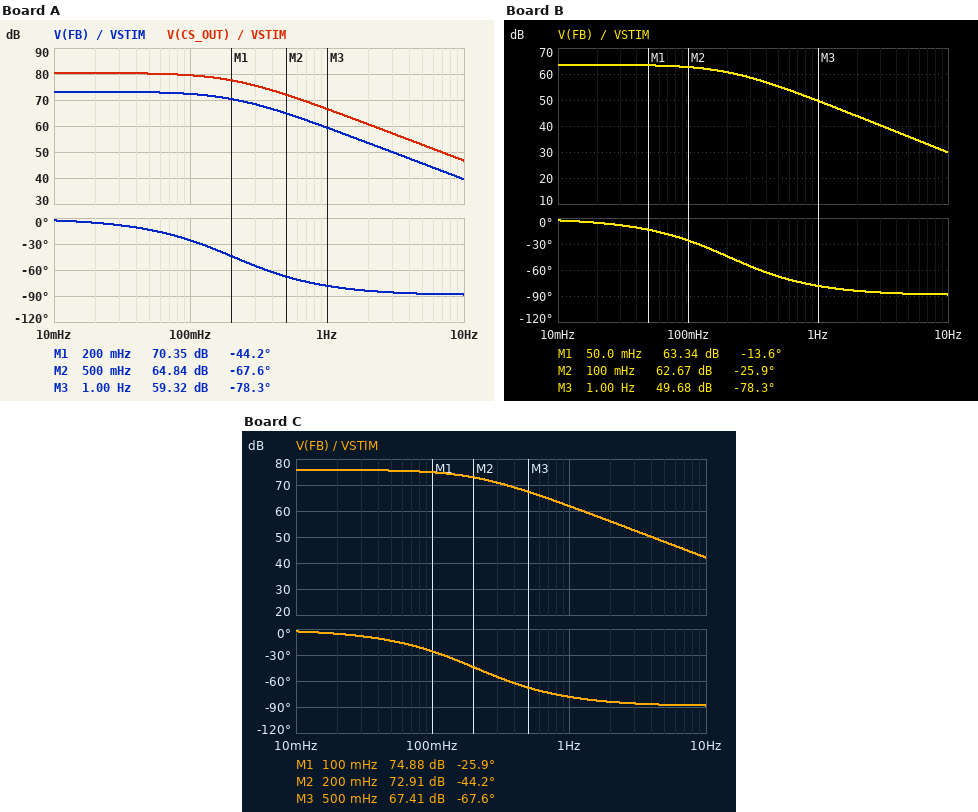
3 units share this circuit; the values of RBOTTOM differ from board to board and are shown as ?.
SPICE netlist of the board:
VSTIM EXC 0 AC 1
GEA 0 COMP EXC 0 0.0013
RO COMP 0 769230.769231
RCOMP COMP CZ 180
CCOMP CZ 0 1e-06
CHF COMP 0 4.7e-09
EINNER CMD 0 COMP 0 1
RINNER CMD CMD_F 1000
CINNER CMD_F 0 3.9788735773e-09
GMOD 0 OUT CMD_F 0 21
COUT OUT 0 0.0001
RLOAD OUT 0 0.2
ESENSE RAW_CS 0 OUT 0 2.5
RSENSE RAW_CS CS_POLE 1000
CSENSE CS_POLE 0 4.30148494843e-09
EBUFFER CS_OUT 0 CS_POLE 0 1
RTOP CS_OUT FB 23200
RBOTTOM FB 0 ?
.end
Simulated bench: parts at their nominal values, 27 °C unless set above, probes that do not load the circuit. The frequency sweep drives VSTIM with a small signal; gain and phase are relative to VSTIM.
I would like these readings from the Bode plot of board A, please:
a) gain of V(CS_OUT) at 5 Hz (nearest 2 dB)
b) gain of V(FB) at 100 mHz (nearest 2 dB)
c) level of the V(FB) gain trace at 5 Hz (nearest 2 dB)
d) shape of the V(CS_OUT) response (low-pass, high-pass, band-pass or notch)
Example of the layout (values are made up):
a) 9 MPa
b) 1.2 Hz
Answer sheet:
a) 52 dB
b) 72 dB
c) 46 dB
d) low-pass
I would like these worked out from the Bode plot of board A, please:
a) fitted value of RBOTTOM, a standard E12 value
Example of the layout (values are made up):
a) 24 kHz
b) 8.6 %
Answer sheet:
a) 18 kΩ
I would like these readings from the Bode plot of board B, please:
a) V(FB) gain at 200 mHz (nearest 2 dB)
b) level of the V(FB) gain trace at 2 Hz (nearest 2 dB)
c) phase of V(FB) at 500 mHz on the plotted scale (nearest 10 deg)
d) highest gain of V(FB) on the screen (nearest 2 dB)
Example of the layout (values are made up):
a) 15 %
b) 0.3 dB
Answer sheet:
a) 60 dB
b) 44 dB
c) -70 deg
d) 64 dB
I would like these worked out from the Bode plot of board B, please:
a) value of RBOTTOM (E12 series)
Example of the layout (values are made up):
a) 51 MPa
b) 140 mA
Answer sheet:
a) 3.9 kΩ
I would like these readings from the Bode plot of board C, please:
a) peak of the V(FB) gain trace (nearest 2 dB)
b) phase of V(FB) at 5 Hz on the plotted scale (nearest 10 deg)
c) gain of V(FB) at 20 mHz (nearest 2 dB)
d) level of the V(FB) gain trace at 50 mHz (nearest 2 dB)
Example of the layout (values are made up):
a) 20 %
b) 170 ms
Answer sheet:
a) 76 dB
b) -90 deg
c) 76 dB
d) 76 dB
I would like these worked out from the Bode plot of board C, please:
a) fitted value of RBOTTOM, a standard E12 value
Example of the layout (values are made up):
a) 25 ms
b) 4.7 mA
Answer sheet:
a) 33 kΩ
